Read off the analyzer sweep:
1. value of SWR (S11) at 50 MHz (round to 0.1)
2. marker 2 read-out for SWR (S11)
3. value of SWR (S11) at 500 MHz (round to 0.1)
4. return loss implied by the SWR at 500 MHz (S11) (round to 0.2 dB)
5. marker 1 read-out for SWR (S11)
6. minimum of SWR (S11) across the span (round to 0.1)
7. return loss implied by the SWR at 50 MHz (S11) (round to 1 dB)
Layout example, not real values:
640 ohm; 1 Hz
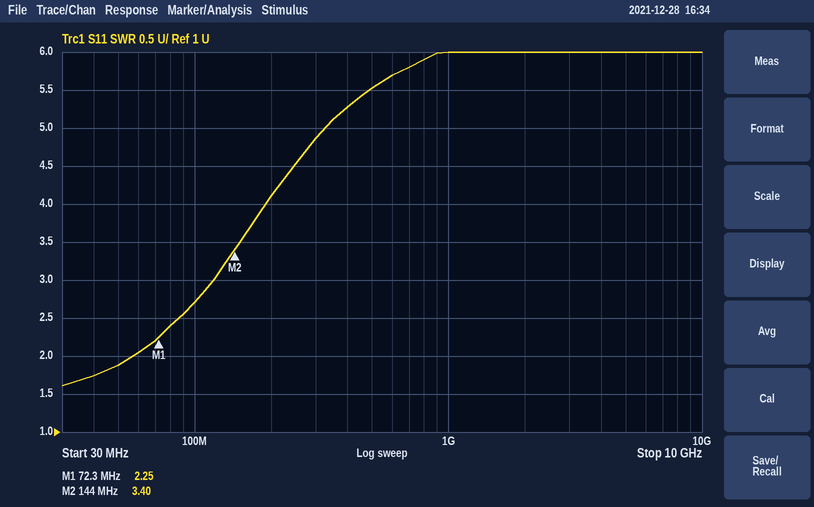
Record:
1.9; 3.40; 5.5; 3.2 dB; 2.25; 1.6; 10 dB
